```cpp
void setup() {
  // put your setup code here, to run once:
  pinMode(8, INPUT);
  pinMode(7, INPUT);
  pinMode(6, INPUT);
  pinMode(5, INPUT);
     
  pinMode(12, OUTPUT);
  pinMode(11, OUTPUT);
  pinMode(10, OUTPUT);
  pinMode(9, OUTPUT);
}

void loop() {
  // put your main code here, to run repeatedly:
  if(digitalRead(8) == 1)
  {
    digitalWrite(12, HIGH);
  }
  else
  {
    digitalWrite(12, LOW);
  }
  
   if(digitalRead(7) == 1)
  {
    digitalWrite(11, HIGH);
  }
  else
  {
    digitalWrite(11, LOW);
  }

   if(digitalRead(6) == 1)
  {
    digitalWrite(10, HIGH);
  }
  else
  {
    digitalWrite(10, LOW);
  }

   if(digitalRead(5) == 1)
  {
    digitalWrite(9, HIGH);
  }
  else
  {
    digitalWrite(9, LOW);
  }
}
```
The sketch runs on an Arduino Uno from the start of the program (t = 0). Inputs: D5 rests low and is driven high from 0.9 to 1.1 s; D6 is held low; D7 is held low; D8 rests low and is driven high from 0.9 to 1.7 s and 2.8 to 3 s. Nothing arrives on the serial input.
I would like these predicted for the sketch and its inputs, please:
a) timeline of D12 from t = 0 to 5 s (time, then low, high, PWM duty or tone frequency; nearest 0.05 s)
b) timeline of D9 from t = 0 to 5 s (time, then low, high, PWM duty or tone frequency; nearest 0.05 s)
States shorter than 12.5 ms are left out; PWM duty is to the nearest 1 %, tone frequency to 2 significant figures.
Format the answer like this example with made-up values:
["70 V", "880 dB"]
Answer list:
["0 s low; 0.9 s high; 1.7 s low; 2.8 s high; 3 s low", "0 s low; 0.9 s high; 1.1 s low"]
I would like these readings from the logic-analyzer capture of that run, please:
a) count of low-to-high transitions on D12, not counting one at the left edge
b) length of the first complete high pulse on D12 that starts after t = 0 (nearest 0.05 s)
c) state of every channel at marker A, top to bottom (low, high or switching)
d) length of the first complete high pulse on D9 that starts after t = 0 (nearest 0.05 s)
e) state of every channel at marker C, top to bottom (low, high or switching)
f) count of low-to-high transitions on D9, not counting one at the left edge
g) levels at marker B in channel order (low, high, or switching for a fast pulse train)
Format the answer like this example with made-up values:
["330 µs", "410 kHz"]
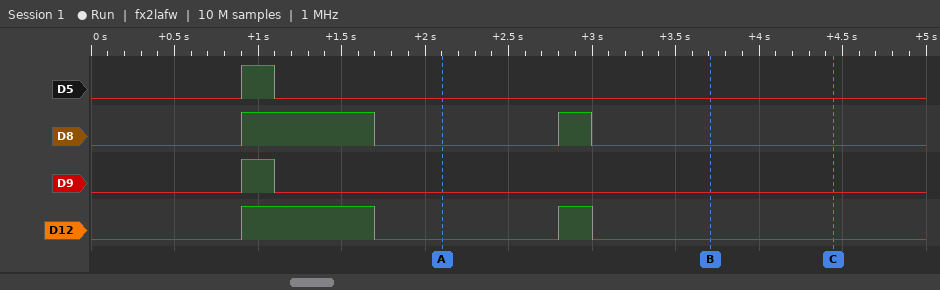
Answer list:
["2", "0.80 s", "D5 low, D8 low, D9 low, D12 low", "0.20 s", "D5 low, D8 low, D9 low, D12 low", "1", "D5 low, D8 low, D9 low, D12 low"]
